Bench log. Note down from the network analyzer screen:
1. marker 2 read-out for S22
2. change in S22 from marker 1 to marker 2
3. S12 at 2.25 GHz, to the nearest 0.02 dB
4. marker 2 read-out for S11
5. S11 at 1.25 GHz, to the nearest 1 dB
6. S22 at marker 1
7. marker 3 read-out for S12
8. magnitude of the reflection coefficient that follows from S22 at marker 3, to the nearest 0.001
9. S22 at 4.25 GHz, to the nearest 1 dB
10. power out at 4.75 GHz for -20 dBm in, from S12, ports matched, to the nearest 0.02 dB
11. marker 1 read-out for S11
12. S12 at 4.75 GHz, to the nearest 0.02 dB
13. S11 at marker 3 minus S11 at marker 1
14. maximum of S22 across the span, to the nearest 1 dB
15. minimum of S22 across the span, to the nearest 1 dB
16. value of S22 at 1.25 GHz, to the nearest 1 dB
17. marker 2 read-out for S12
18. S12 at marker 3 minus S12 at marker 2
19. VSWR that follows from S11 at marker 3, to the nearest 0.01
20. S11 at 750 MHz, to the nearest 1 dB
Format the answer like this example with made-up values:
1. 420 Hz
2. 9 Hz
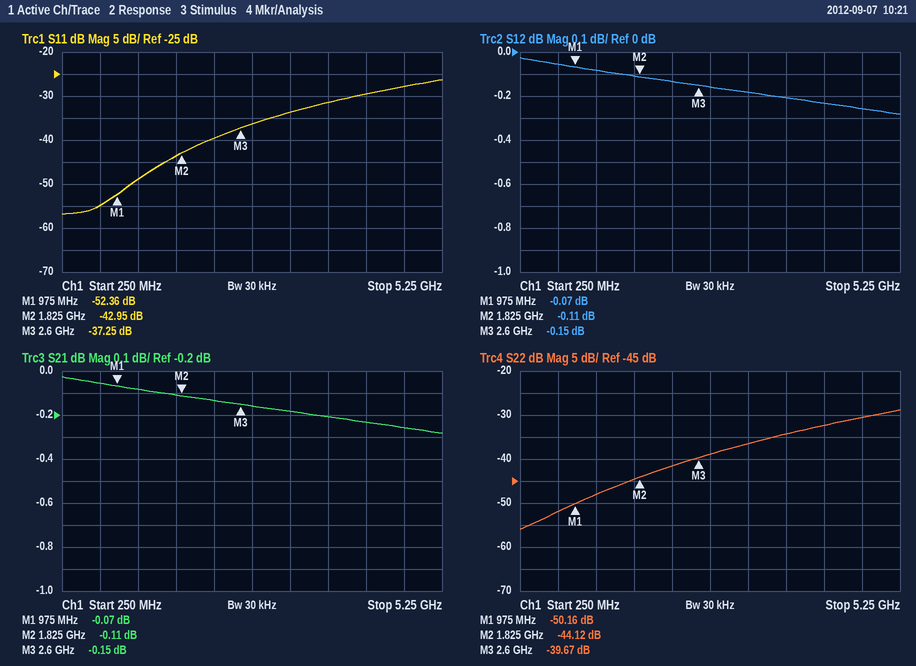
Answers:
1. -44.12 dB
2. 6.04 dB
3. -0.14 dB
4. -42.95 dB
5. -49 dB
6. -50.16 dB
7. -0.15 dB
8. 0.010
9. -32 dB
10. -20.26 dBm
11. -52.36 dB
12. -0.26 dB
13. 15.11 dB
14. -29 dB
15. -56 dB
16. -48 dB
17. -0.11 dB
18. -0.04 dB
19. 1.03
20. -55 dB
